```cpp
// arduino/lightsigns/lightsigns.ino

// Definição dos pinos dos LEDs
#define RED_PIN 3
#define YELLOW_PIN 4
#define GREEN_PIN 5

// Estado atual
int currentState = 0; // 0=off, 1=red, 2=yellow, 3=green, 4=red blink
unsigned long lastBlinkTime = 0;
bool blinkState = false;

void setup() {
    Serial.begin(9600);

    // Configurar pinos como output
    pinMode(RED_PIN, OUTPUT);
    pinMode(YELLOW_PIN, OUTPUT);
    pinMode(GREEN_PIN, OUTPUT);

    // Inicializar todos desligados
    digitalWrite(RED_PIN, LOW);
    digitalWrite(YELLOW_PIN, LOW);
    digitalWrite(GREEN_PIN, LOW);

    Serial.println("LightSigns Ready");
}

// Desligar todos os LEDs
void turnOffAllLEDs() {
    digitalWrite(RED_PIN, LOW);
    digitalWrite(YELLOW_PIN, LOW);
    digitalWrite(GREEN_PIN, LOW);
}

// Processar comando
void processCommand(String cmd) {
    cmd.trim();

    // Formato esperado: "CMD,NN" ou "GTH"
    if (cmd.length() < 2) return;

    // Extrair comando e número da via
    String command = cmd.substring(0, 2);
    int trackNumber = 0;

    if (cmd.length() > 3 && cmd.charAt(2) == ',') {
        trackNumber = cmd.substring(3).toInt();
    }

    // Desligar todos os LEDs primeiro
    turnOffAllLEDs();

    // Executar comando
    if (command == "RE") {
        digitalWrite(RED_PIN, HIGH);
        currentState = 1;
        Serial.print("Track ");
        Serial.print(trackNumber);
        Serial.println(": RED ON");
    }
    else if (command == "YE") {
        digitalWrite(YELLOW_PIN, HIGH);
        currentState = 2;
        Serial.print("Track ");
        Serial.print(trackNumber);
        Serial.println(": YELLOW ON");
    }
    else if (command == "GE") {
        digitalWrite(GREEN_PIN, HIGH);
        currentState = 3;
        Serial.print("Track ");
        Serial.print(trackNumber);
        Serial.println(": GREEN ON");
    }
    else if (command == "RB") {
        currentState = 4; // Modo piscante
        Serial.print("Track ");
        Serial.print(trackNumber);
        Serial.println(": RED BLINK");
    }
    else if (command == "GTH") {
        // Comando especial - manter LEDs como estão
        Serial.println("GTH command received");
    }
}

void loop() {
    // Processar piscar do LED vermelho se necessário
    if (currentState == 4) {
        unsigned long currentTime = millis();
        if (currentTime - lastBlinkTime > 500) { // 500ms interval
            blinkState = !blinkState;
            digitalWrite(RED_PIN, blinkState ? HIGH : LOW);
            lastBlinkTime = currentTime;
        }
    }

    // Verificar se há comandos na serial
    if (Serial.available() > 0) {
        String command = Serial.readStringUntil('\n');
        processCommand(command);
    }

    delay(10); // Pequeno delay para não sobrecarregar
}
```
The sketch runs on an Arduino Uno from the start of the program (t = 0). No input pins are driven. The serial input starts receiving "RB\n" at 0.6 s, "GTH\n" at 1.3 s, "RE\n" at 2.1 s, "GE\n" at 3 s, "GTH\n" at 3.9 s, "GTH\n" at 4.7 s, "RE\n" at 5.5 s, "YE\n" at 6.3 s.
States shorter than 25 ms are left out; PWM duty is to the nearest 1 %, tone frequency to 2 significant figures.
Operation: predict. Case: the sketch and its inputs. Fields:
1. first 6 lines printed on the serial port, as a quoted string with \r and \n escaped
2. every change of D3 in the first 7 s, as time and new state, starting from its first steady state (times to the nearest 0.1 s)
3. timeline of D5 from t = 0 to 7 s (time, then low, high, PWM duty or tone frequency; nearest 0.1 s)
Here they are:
"LightSigns Ready\r\nTrack 0: RED BLINK\r\nTrack 0: RED ON\r\nTrack 0: GREEN ON\r\nTrack 0: RED ON\r\nTrack 0: YELLOW ON\r\n"
0 s low; 0.6 s high; 1.1 s low; 1.6 s high; 3 s low; 5.5 s high; 6.3 s low
0 s low; 3 s high; 3.9 s low
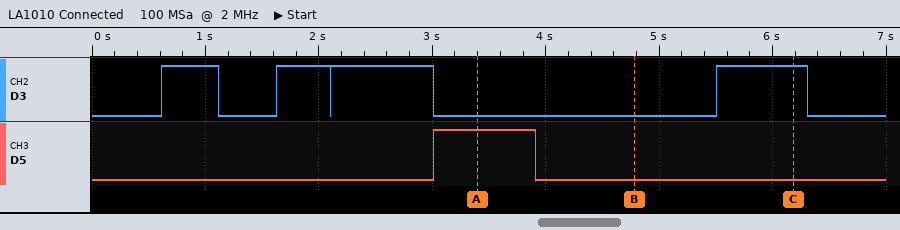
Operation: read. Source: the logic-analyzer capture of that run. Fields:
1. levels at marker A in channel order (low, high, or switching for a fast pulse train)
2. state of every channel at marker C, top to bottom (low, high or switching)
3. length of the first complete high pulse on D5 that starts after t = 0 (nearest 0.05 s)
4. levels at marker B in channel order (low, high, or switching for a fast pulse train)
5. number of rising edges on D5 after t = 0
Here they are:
D3 low, D5 high
D3 high, D5 low
0.90 s
D3 low, D5 low
1
